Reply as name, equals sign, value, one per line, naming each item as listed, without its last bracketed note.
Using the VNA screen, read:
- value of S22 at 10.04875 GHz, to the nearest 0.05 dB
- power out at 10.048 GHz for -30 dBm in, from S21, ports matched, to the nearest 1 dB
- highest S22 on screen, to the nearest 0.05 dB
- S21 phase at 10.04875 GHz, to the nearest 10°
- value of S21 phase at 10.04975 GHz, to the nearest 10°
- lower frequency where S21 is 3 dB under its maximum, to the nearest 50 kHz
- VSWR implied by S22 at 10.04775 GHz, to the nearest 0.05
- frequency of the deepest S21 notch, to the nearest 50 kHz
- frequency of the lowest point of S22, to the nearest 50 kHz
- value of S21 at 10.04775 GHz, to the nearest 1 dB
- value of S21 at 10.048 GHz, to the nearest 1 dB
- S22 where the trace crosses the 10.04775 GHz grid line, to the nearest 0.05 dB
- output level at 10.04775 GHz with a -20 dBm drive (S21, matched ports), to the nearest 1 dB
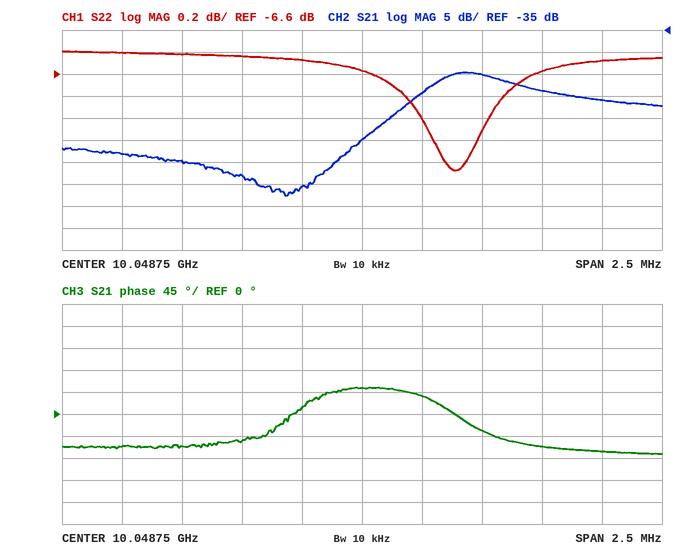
value of S22 at 10.04875 GHz, to the nearest 0.05 dB = -6.55 dB
power out at 10.048 GHz for -30 dBm in, from S21, ports matched, to the nearest 1 dB = -95 dBm
highest S22 on screen, to the nearest 0.05 dB = -6.40 dB
S21 phase at 10.04875 GHz, to the nearest 10° = 50°
value of S21 phase at 10.04975 GHz, to the nearest 10° = -80°
lower frequency where S21 is 3 dB under its maximum, to the nearest 50 kHz = 10.04905 GHz
VSWR implied by S22 at 10.04775 GHz, to the nearest 0.05 = 2.85
frequency of the deepest S21 notch, to the nearest 50 kHz = 10.04845 GHz
frequency of the lowest point of S22, to the nearest 50 kHz = 10.04915 GHz
value of S21 at 10.04775 GHz, to the nearest 1 dB = -63 dB
value of S21 at 10.048 GHz, to the nearest 1 dB = -65 dB
S22 where the trace crosses the 10.04775 GHz grid line, to the nearest 0.05 dB = -6.40 dB
output level at 10.04775 GHz with a -20 dBm drive (S21, matched ports), to the nearest 1 dB = -83 dBm
